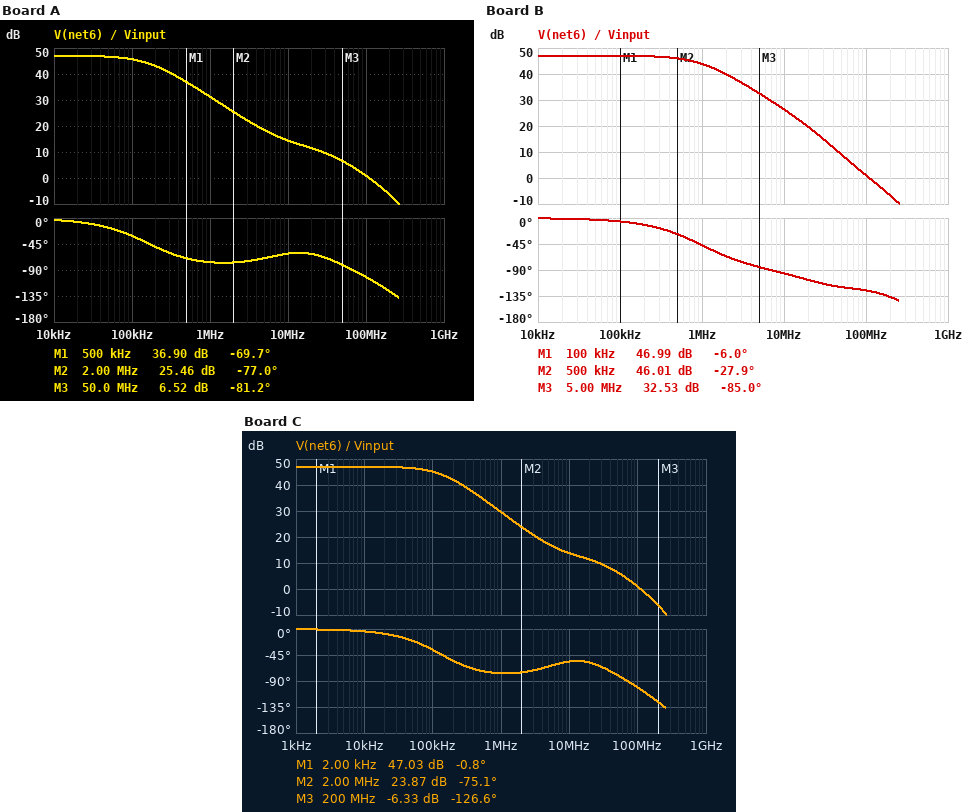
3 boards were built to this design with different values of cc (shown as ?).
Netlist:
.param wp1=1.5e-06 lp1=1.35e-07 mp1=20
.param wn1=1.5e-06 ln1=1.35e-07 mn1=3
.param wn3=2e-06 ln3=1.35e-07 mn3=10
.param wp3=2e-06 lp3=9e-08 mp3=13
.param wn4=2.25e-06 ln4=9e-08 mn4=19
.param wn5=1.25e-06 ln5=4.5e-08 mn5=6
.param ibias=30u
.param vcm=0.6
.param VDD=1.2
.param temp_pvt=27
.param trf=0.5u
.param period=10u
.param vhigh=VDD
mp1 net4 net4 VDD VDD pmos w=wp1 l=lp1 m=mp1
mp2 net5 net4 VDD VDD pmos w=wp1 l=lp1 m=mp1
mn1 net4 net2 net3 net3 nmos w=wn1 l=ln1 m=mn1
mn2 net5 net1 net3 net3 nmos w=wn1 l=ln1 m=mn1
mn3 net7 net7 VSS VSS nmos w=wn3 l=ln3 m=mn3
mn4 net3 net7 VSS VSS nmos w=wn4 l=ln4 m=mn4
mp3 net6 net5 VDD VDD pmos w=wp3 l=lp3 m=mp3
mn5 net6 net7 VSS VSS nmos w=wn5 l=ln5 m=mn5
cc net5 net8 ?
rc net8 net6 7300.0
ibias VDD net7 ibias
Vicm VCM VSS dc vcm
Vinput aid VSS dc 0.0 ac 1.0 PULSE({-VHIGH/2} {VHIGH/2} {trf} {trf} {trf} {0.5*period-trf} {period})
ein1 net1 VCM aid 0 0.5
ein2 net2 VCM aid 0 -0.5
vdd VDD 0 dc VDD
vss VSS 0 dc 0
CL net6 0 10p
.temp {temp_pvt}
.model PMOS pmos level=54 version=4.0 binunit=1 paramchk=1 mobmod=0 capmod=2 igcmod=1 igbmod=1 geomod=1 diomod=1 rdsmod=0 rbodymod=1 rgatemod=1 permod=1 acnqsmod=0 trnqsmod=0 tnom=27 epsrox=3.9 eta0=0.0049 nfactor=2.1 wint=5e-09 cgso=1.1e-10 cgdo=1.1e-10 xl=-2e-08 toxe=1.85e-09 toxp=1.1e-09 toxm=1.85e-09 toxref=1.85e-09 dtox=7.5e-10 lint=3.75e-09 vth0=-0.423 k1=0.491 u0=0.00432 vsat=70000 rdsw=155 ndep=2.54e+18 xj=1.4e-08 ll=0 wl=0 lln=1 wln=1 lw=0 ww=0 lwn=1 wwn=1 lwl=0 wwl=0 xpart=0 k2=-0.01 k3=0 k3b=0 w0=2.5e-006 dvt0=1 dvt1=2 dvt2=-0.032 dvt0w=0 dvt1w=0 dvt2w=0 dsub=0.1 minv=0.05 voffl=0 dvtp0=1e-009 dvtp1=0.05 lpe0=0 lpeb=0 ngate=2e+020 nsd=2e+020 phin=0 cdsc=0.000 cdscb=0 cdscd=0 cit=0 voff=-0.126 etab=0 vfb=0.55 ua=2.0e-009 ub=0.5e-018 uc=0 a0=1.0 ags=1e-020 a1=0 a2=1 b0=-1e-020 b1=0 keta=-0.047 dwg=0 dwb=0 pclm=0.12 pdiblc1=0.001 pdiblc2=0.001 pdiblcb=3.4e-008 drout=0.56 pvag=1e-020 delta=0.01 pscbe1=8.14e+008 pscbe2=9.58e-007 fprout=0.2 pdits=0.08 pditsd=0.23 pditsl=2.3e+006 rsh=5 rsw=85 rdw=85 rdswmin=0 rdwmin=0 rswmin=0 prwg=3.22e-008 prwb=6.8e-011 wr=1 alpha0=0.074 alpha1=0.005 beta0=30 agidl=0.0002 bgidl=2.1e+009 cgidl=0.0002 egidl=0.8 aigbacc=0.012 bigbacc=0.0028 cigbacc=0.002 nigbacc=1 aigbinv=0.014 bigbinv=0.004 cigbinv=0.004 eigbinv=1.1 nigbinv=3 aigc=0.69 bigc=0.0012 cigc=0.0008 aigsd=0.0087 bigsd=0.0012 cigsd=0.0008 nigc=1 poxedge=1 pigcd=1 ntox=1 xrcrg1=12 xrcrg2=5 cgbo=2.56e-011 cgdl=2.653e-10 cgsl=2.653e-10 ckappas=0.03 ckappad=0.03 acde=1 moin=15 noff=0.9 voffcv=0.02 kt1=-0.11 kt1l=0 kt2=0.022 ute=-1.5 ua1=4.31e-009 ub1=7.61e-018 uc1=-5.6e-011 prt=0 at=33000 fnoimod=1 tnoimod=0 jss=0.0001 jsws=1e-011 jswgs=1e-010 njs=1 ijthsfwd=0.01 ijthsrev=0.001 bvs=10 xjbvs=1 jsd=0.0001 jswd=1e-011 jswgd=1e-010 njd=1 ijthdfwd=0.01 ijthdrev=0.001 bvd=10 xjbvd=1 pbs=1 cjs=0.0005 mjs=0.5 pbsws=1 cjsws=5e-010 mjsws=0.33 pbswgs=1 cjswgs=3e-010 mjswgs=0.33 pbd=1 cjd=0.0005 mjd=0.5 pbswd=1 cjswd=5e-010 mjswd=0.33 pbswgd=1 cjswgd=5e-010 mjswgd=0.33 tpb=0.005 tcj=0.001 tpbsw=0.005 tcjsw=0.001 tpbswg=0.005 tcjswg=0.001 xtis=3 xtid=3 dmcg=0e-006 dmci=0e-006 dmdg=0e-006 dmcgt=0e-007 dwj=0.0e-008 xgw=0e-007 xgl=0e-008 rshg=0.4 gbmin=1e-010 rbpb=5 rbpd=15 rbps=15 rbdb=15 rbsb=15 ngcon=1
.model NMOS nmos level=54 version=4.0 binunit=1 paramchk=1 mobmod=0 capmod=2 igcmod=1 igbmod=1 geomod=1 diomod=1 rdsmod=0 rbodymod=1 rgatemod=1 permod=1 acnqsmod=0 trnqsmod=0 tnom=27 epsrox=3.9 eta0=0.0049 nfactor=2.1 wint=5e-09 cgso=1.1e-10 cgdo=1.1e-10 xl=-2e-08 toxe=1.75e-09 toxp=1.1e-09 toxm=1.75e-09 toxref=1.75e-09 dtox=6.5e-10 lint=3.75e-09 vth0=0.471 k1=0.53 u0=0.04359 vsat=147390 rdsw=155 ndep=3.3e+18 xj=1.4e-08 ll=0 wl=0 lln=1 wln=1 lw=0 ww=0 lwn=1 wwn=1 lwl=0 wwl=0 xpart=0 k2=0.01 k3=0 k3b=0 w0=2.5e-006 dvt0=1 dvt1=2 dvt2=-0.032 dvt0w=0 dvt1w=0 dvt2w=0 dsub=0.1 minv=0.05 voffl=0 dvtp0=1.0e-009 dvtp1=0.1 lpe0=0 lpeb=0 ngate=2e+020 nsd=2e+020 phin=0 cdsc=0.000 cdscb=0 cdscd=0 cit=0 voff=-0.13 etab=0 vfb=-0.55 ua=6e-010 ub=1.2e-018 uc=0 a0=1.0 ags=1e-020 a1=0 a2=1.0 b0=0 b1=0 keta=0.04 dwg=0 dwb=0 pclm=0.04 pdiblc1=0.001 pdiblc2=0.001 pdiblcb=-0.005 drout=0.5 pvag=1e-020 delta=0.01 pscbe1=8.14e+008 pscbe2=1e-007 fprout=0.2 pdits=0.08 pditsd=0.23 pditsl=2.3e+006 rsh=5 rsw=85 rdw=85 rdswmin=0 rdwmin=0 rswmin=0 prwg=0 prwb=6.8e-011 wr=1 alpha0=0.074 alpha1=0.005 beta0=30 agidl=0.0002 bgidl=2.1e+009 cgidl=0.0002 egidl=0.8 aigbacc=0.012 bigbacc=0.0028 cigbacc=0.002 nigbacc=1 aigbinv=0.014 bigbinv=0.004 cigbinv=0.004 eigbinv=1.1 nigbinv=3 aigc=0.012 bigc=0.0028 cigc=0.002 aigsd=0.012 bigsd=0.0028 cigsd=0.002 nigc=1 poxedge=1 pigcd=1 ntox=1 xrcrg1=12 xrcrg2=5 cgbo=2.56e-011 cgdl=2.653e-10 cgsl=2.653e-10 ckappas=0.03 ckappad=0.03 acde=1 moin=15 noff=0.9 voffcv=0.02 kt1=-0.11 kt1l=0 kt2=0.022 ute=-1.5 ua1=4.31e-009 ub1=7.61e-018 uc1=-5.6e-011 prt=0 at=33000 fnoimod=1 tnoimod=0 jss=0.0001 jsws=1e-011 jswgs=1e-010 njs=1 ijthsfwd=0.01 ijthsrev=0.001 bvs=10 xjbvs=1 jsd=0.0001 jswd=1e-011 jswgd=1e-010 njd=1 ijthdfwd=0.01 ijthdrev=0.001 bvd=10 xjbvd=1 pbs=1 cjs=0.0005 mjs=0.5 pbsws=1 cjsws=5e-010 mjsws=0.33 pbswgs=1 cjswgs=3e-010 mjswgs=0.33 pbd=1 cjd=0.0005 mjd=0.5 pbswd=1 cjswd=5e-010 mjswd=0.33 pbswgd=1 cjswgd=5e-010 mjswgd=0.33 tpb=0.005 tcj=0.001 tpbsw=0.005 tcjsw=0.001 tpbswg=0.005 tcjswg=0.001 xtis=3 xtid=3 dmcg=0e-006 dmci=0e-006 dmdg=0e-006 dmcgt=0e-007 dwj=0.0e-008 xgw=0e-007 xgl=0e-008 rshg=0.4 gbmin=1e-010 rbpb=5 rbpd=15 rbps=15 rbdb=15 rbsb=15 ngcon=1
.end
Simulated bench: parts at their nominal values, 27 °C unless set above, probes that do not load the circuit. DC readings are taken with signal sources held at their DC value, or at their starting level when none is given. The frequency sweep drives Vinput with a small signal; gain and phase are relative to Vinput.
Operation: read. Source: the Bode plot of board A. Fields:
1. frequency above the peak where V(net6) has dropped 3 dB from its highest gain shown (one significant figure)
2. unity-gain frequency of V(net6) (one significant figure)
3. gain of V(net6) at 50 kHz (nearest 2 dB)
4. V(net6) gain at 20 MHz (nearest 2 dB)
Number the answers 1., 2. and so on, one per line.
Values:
1. 200 kHz
2. 100 MHz
3. 46 dB
4. 12 dB
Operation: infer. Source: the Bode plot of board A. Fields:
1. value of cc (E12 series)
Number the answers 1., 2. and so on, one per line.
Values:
1. 2.7 pF
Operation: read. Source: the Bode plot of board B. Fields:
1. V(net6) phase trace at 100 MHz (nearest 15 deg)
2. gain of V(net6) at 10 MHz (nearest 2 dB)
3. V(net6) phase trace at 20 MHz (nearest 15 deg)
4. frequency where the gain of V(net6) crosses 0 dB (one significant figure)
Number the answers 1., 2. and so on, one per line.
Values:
1. -120 deg
2. 26 dB
3. -105 deg
4. 100 MHz
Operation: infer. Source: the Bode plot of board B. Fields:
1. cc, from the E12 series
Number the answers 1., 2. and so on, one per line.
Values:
1. 390 fF
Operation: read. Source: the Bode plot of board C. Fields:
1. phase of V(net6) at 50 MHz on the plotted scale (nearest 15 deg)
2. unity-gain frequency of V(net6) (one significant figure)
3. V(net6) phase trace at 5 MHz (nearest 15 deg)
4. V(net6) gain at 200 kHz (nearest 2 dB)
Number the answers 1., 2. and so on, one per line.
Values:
1. -75 deg
2. 100 MHz
3. -60 deg
4. 42 dB
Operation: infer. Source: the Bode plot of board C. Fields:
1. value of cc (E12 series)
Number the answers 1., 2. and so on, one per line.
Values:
1. 3.3 pF
